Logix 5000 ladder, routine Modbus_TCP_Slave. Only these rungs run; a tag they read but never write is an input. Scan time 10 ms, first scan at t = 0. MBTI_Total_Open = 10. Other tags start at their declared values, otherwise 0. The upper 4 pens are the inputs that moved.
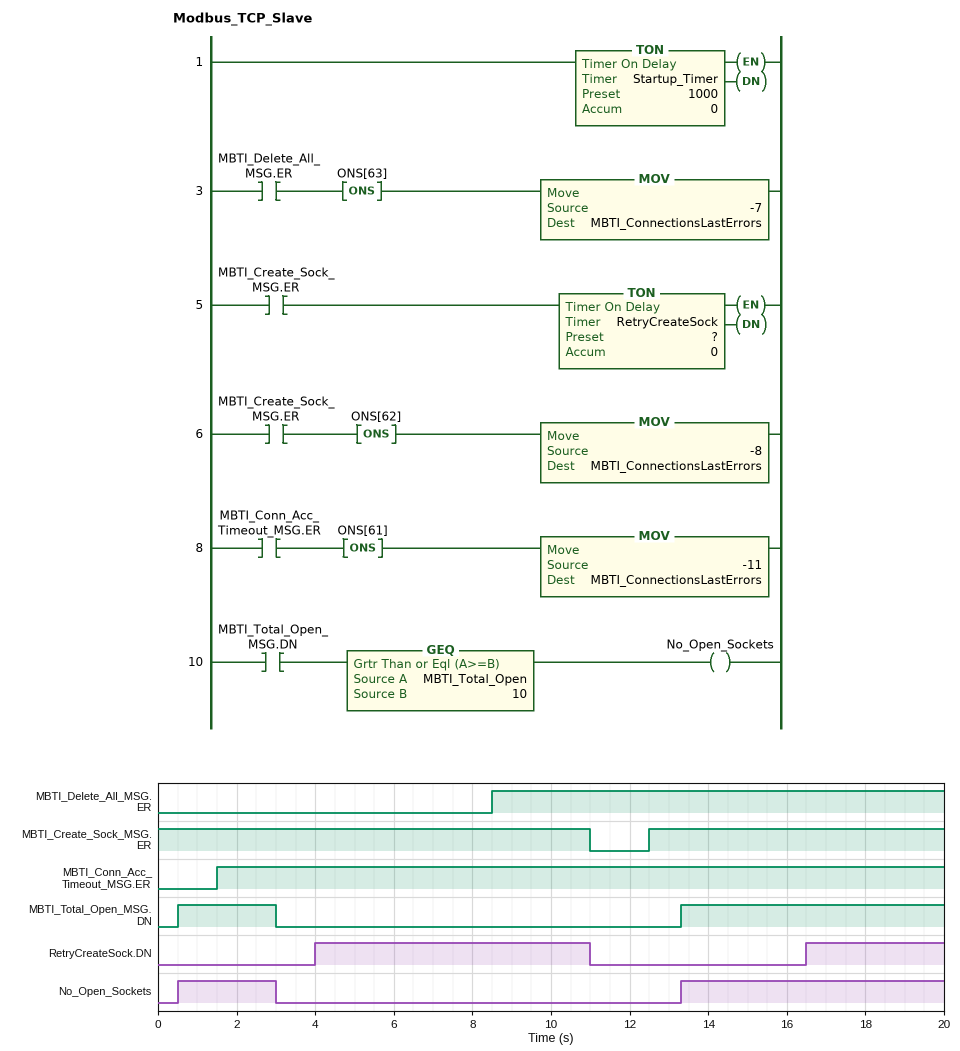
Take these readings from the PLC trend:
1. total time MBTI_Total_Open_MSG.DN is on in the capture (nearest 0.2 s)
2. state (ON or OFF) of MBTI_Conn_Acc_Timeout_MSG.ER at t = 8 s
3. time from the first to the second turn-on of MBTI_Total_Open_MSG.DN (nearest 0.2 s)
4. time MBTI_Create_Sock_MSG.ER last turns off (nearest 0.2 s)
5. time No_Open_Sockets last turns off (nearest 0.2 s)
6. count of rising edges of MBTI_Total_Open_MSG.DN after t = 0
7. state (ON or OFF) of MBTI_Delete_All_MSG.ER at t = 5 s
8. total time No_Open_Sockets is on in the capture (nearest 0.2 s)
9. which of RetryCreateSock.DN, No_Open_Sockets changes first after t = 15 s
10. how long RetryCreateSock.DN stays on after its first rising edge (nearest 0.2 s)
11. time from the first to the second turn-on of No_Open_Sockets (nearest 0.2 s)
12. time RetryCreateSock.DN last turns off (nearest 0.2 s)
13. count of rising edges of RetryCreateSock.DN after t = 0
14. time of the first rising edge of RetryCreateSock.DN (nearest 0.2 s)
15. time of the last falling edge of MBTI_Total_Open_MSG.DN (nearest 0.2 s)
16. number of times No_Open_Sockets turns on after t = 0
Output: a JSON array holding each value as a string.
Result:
["9.2 s", "ON", "12.8 s", "11.0 s", "3.0 s", "2", "OFF", "9.2 s", "RetryCreateSock.DN", "7.0 s", "12.8 s", "11.0 s", "2", "4.0 s", "3.0 s", "2"]
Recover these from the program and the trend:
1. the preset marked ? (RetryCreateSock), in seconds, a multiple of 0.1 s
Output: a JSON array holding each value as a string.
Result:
["4.0 s"]
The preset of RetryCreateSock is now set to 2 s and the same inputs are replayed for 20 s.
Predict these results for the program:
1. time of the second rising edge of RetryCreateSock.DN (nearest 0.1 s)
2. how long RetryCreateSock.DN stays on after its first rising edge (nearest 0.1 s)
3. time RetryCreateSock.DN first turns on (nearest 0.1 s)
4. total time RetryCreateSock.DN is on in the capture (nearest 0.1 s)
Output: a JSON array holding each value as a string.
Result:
["14.5 s", "9.0 s", "2.0 s", "14.5 s"]
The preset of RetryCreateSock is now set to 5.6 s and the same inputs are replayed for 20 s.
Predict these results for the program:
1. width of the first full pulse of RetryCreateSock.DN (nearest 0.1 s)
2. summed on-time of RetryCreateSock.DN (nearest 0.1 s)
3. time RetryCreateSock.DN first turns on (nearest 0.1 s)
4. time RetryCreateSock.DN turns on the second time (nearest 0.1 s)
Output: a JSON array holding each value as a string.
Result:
["5.4 s", "7.3 s", "5.6 s", "18.1 s"]
